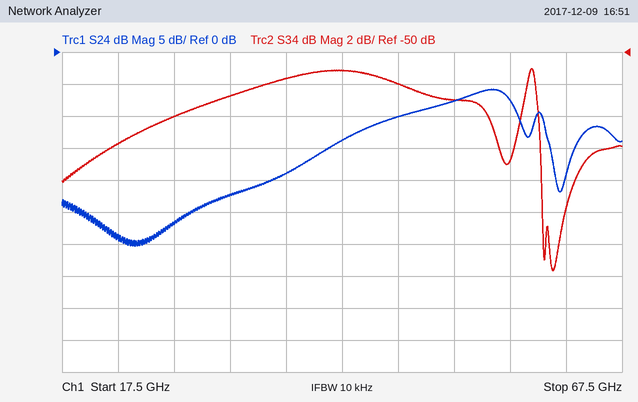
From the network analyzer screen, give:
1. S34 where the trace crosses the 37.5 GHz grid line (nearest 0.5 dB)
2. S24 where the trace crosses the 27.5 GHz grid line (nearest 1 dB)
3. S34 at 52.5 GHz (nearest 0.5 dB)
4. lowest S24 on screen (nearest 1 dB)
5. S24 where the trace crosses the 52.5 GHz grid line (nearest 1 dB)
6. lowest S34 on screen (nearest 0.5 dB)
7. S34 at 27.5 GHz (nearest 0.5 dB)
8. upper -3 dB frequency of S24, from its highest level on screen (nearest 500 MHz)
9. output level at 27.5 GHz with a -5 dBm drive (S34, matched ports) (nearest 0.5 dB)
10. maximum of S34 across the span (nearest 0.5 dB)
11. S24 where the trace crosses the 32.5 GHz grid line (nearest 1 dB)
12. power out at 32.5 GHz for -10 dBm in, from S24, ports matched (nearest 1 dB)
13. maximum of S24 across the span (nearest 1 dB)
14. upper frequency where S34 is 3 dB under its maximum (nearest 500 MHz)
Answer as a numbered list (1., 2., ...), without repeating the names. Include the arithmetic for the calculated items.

1. -51.5 dB
2. -27 dB
3. -53.0 dB
4. -30 dB
5. -8 dB
6. -63.5 dB
7. -54.0 dB
8. 58.0 GHz
9. -5 dBm + (-54.0 dB) = -59.0 dBm
10. -51.0 dB
11. -22 dB
12. -10 dBm + (-22 dB) = -32 dBm
13. -6 dB
14. 60.0 GHz
